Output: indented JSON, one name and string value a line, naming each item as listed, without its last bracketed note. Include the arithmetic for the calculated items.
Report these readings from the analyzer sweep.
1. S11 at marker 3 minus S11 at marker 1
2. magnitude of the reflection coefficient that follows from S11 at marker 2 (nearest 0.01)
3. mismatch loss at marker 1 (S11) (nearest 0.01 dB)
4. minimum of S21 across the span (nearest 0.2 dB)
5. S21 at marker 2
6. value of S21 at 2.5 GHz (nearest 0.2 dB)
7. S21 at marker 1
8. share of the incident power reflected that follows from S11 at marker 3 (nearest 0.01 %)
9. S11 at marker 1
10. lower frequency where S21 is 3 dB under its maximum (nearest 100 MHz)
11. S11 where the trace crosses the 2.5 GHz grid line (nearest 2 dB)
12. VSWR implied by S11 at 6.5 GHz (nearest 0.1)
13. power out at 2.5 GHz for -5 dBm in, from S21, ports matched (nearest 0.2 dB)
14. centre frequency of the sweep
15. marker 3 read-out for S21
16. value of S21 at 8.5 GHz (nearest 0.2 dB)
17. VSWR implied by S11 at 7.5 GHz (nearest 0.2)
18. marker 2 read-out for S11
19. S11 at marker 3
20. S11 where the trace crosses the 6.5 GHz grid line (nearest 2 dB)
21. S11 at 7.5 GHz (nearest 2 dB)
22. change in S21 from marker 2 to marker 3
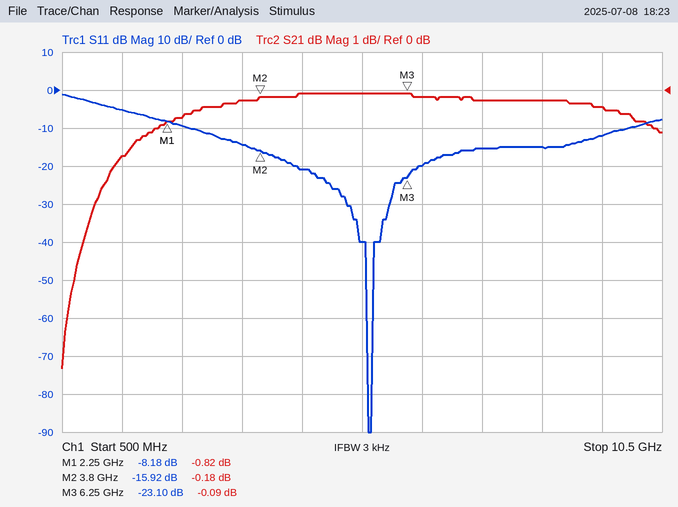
{
  "S11 at marker 3 minus S11 at marker 1": "-23.1 − (-8.18) = -14.92 dB",
  "magnitude of the reflection coefficient that follows from S11 at marker 2": "10^(-15.92/20) ≈ 0.16",
  "mismatch loss at marker 1 (S11)": "−10 log10(1 − 10^(-8.18/10)) ≈ 0.72 dB",
  "minimum of S21 across the span": "-7.4 dB",
  "S21 at marker 2": "-0.18 dB",
  "value of S21 at 2.5 GHz": "-0.8 dB",
  "S21 at marker 1": "-0.82 dB",
  "share of the incident power reflected that follows from S11 at marker 3": "10^(-23.1/10) ≈ 0.49 %",
  "S11 at marker 1": "-8.18 dB",
  "lower frequency where S21 is 3 dB under its maximum": "1.0 GHz",
  "S11 where the trace crosses the 2.5 GHz grid line": "-10 dB",
  "VSWR implied by S11 at 6.5 GHz": "|Γ| = 10^(-20/20) = 0.1000; VSWR = (1 + 0.1000)/(1 − 0.1000) ≈ 1.2",
  "power out at 2.5 GHz for -5 dBm in, from S21, ports matched": "-5 dBm + (-0.8 dB) = -5.8 dBm",
  "centre frequency of the sweep": "5.5 GHz",
  "marker 3 read-out for S21": "-0.09 dB",
  "value of S21 at 8.5 GHz": "-0.2 dB",
  "VSWR implied by S11 at 7.5 GHz": "|Γ| = 10^(-16/20) = 0.1585; VSWR = (1 + 0.1585)/(1 − 0.1585) ≈ 1.4",
  "marker 2 read-out for S11": "-15.92 dB",
  "S11 at marker 3": "-23.10 dB",
  "S11 where the trace crosses the 6.5 GHz grid line": "-20 dB",
  "S11 at 7.5 GHz": "-16 dB",
  "change in S21 from marker 2 to marker 3": "-0.09 − (-0.18) = 0.09 dB"
}
